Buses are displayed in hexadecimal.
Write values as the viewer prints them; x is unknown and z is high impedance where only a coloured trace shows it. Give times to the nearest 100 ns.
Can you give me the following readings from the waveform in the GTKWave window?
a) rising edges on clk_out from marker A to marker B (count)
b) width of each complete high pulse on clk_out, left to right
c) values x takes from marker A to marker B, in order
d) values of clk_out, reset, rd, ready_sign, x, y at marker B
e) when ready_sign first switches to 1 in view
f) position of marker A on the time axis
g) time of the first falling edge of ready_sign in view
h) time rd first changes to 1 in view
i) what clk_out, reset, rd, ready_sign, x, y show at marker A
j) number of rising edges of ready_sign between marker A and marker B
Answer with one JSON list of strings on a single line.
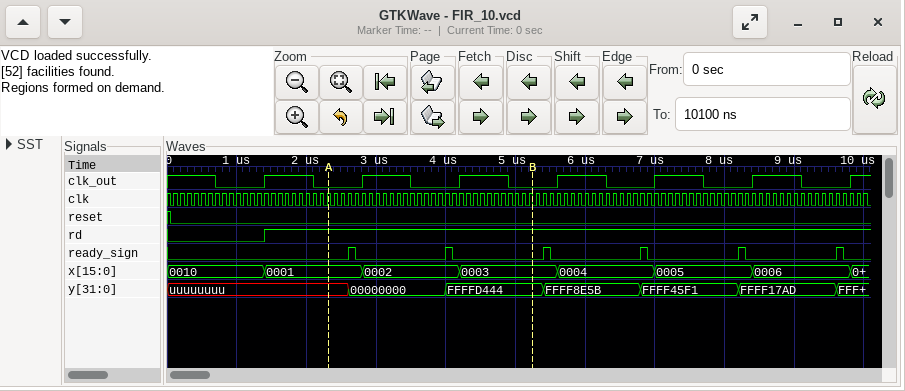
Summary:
["2", "700 ns, 700 ns, 700 ns, 700 ns, 700 ns, 700 ns", "0001, 0002, 0003", "clk_out=0, reset=0, rd=1, ready_sign=0, x=0003, y=FFFFD444", "2600 ns", "2300 ns", "2700 ns", "1400 ns", "clk_out=0, reset=0, rd=1, ready_sign=0, x=0001, y=uuuuuuuu", "2"]
